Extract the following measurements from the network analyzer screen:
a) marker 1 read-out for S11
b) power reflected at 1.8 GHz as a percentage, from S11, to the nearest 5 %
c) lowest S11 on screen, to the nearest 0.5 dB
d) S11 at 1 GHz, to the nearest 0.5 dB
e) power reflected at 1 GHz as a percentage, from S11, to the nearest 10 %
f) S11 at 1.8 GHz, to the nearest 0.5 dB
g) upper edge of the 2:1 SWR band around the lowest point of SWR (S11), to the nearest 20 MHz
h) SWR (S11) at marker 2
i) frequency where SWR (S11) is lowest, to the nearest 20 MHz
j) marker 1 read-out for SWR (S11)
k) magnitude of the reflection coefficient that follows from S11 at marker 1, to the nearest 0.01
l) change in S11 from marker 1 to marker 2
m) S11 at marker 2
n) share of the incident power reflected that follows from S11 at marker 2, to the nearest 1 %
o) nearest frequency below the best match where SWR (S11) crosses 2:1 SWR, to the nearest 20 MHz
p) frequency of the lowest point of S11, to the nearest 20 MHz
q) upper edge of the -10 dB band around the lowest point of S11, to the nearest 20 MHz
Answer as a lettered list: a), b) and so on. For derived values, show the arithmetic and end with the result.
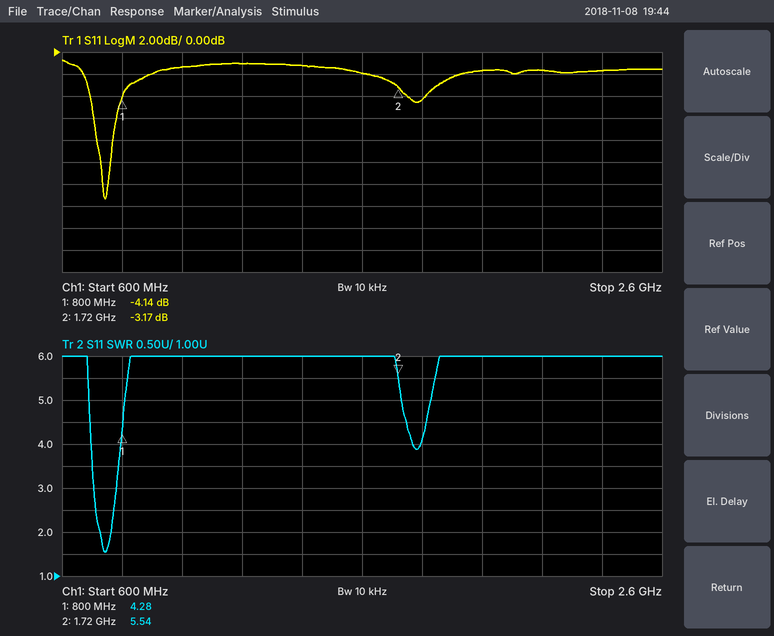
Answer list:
a) -4.14 dB
b) 10^(-4.5/10) ≈ 35 %
c) -13.5 dB
d) -1.5 dB
e) 10^(-1.5/10) ≈ 70.8 %, so 70 % to the nearest 10 %
f) -4.5 dB
g) 760 MHz
h) 5.54
i) 740 MHz
j) 4.28
k) 10^(-4.14/20) ≈ 0.62
l) -3.17 − (-4.14) = 0.97 dB
m) -3.17 dB
n) 10^(-3.17/10) ≈ 48 %
o) 720 MHz
p) 740 MHz
q) 760 MHz
